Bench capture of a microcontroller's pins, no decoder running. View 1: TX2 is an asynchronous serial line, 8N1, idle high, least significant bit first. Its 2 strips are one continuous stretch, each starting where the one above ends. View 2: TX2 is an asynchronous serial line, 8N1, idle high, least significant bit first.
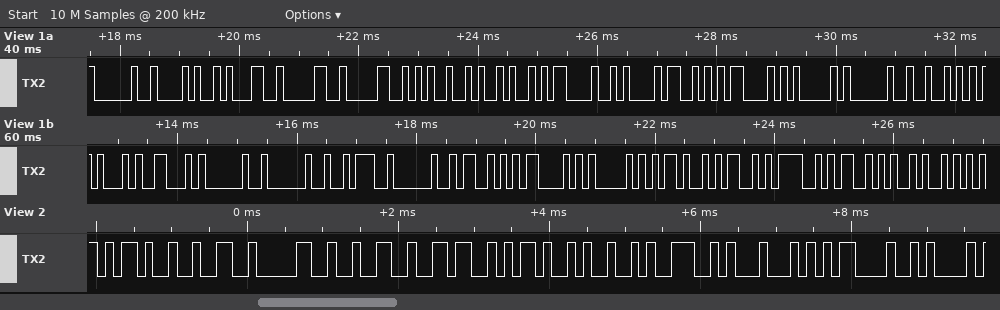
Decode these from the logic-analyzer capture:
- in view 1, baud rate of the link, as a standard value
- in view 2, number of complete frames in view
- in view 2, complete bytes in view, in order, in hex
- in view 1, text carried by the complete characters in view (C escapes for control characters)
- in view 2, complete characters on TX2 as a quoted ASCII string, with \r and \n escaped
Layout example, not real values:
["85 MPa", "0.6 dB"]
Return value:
["9600 baud", "11", "2D 32 30 32 36 2D 49 4E 44 0D 0A", "\" (100%)\\r\\nSCA REF  : SCA-MOSJ\"", "\"-2026-IND\\r\\n\""]
